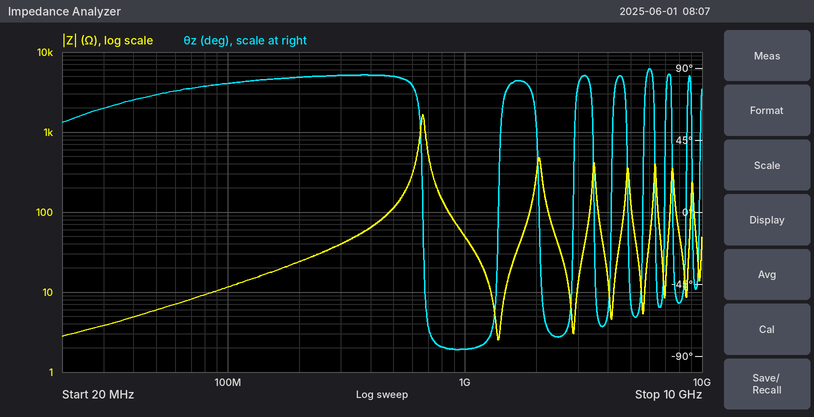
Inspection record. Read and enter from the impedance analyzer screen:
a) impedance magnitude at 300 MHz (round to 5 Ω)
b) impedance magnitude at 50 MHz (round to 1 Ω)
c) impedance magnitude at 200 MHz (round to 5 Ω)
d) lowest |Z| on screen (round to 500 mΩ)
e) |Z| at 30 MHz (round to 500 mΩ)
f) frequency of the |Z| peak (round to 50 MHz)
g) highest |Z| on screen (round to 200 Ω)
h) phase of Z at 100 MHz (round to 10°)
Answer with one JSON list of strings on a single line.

["40 Ω", "6 Ω", "25 Ω", "2.5 Ω", "4.0 Ω", "650 MHz", "1.6 kΩ", "80°"]
